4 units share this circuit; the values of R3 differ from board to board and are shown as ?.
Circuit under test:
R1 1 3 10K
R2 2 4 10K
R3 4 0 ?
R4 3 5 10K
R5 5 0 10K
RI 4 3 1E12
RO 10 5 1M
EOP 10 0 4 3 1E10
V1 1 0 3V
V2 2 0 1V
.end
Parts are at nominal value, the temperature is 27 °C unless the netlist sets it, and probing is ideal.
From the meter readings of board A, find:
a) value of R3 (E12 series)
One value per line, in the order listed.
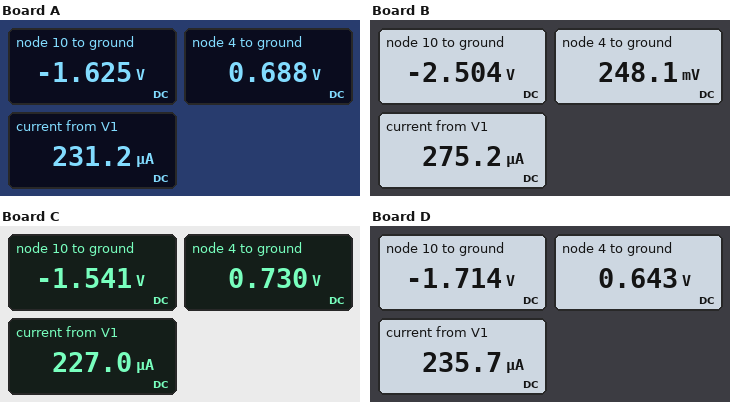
22 kΩ
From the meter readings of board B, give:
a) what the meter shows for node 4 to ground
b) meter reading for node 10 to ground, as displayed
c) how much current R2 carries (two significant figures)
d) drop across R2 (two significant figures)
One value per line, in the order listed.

248.1 mV
-2.504 V
75 µA
750 mV
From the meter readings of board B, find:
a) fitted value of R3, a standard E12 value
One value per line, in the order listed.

3.3 kΩ
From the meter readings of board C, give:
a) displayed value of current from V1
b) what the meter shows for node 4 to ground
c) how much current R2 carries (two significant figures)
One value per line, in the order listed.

227.0 µA
0.730 V
27 µA
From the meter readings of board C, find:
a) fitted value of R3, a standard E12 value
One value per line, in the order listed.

27 kΩ
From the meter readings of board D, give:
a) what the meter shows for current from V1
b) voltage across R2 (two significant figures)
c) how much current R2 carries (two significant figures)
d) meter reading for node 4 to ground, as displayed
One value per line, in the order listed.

235.7 µA
360 mV
36 µA
0.643 V
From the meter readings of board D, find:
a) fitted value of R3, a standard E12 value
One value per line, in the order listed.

18 kΩ
